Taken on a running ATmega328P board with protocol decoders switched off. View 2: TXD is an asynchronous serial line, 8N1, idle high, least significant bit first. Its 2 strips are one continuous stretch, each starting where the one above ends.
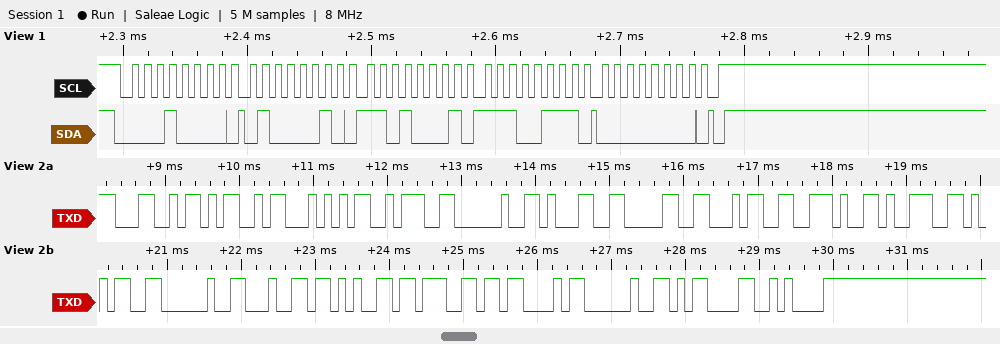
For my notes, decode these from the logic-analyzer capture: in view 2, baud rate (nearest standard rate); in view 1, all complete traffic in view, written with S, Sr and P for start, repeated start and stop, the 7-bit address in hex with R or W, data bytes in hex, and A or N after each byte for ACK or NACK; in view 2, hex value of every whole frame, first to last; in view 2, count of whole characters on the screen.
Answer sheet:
9600 baud
S 08W A 42 A D1 A E7 A 00 A P
4C 4D 54 3A 20 31 30 34 2E 39 35 20 64 65 67 43 20 0D 0A
19
